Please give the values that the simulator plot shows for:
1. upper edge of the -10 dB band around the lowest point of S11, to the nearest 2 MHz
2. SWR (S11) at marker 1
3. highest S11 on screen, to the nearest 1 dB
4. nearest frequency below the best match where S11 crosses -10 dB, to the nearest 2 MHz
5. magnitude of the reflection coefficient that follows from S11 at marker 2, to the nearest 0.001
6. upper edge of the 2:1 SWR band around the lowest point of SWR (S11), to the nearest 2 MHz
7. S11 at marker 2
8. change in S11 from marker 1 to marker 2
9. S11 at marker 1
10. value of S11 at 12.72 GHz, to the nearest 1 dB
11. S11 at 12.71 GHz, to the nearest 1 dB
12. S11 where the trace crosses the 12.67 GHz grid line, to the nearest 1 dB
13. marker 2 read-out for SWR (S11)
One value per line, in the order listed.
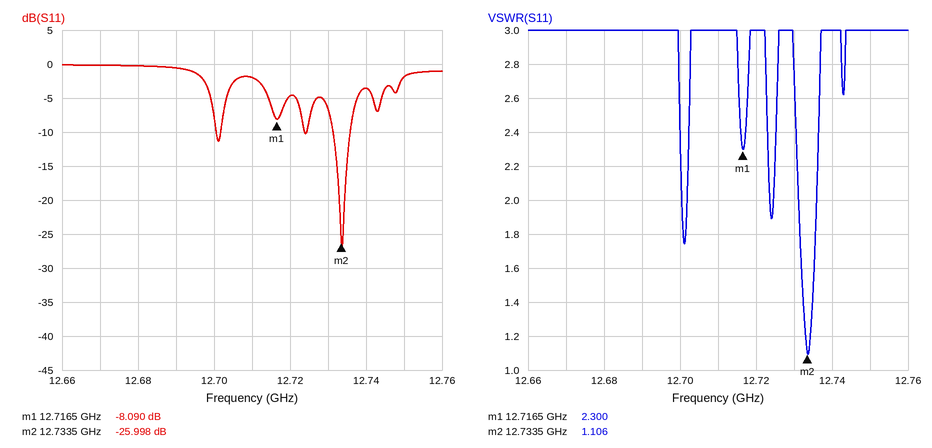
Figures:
12.736 GHz
2.300
0 dB
12.732 GHz
0.050
12.736 GHz
-25.998 dB
-17.908 dB
-8.090 dB
-5 dB
-2 dB
0 dB
1.106
